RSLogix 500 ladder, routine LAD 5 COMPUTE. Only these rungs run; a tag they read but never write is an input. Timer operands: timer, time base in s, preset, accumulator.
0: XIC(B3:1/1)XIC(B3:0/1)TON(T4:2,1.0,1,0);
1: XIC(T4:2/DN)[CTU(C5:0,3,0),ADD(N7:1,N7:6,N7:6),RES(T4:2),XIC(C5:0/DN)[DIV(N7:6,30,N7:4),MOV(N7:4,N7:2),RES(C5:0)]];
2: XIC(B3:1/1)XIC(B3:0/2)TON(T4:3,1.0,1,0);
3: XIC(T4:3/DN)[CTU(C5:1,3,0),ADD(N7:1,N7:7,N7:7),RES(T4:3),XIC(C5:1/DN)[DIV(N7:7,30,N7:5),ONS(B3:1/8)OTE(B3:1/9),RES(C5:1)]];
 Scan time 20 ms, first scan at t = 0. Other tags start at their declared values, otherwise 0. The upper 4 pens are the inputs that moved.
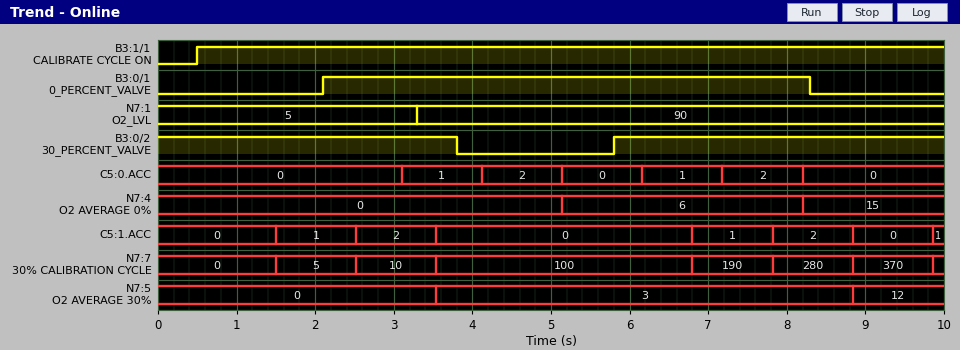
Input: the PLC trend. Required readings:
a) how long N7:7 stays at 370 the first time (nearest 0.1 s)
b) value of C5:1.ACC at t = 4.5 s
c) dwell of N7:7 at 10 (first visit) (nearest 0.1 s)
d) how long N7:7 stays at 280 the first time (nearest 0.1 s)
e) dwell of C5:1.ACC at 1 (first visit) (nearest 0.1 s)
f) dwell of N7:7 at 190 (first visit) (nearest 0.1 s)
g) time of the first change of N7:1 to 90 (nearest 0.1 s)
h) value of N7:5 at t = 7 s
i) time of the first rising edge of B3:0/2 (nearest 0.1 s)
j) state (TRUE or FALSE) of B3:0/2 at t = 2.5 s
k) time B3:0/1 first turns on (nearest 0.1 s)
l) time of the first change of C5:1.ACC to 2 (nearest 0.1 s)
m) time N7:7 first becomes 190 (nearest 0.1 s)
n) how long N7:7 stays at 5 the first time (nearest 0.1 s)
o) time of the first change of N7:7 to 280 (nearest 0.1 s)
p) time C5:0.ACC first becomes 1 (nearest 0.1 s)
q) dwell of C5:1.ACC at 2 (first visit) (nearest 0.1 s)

1.0 s
0
1.0 s
1.0 s
1.0 s
1.0 s
3.3 s
3
5.8 s
TRUE
2.1 s
2.5 s
6.8 s
1.0 s
7.8 s
3.1 s
1.0 s
